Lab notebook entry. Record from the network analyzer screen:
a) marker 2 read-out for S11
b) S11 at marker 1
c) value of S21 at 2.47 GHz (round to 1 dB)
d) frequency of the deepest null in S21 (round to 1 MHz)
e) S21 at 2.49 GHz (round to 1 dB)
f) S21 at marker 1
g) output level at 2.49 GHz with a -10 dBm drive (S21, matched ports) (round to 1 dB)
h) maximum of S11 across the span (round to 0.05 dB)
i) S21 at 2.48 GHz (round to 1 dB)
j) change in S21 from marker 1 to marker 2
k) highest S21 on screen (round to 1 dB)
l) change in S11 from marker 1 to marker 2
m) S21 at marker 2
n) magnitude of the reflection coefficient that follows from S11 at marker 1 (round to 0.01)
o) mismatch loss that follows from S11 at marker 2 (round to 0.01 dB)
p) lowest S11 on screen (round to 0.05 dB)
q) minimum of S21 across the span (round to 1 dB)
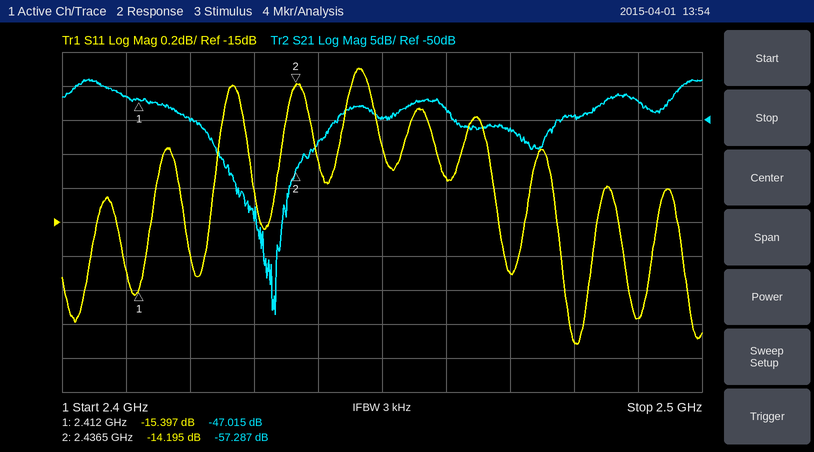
-14.195 dB
-15.397 dB
-51 dB
2.433 GHz
-47 dB
-47.015 dB
-57 dBm
-14.10 dB
-49 dB
-10.272 dB
-44 dB
1.202 dB
-57.287 dB
0.17
0.17 dB
-15.70 dB
-79 dB
